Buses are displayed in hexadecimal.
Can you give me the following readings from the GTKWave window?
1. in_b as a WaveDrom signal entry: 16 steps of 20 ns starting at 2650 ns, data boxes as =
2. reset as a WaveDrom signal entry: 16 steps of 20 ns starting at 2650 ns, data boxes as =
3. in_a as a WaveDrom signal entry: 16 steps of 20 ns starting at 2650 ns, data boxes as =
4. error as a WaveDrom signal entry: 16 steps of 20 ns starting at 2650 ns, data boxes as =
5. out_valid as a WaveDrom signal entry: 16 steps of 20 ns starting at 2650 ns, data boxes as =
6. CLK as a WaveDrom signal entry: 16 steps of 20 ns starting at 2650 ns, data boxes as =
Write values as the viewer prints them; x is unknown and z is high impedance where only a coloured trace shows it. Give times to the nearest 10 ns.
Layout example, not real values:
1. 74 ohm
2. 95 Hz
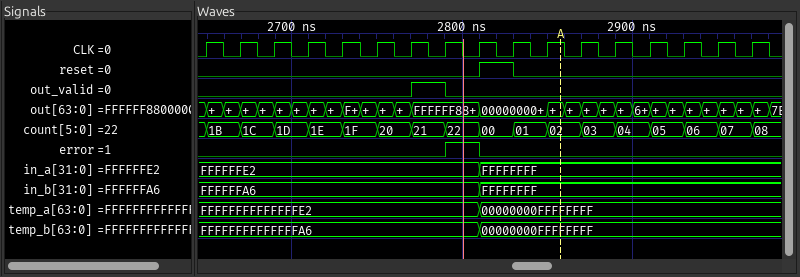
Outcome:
1. {name: 'in_b', wave: '=.......=.......', data: 'FFFFFFA6 FFFFFFFF'}
2. {name: 'reset', wave: '0.......10......'}
3. {name: 'in_a', wave: '=.......=.......', data: 'FFFFFFE2 FFFFFFFF'}
4. {name: 'error', wave: '0......10.......'}
5. {name: 'out_valid', wave: '0.....10........'}
6. {name: 'CLK', wave: 'p...............'}
